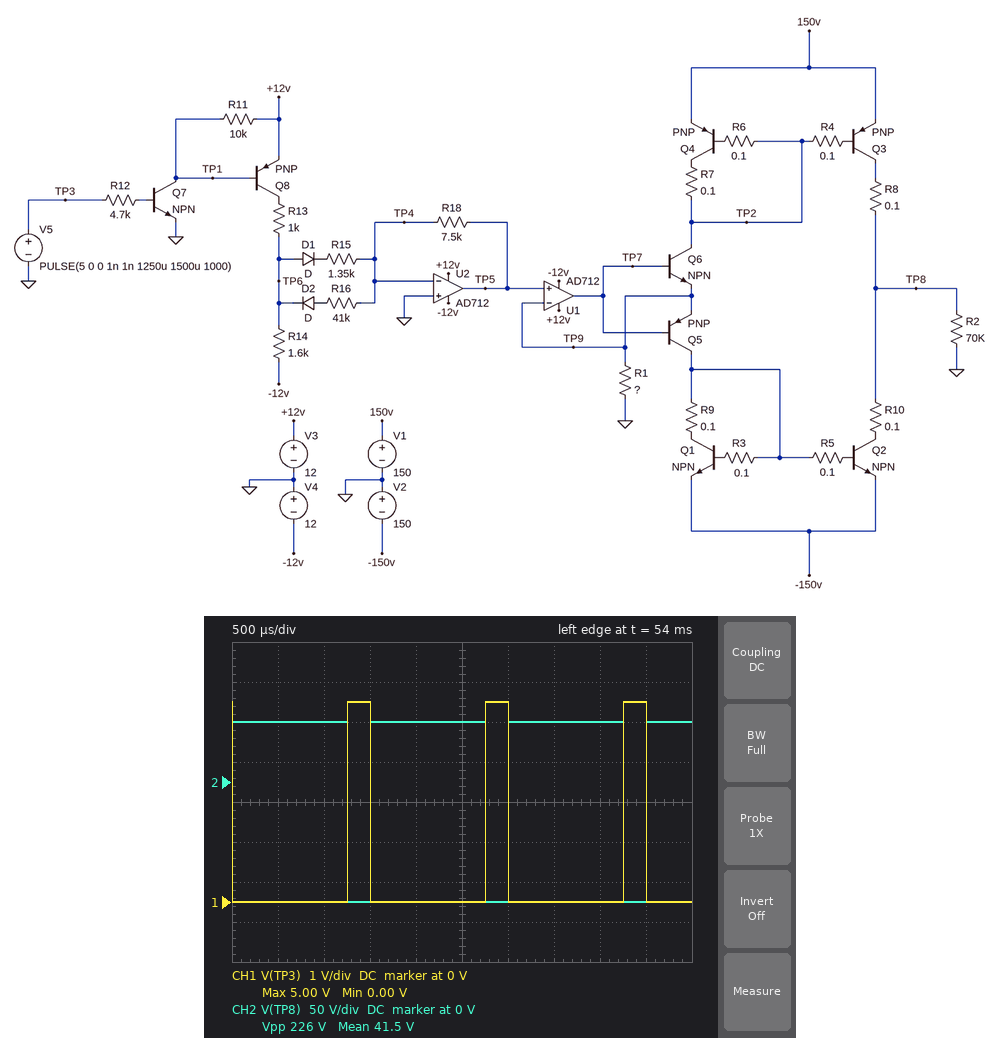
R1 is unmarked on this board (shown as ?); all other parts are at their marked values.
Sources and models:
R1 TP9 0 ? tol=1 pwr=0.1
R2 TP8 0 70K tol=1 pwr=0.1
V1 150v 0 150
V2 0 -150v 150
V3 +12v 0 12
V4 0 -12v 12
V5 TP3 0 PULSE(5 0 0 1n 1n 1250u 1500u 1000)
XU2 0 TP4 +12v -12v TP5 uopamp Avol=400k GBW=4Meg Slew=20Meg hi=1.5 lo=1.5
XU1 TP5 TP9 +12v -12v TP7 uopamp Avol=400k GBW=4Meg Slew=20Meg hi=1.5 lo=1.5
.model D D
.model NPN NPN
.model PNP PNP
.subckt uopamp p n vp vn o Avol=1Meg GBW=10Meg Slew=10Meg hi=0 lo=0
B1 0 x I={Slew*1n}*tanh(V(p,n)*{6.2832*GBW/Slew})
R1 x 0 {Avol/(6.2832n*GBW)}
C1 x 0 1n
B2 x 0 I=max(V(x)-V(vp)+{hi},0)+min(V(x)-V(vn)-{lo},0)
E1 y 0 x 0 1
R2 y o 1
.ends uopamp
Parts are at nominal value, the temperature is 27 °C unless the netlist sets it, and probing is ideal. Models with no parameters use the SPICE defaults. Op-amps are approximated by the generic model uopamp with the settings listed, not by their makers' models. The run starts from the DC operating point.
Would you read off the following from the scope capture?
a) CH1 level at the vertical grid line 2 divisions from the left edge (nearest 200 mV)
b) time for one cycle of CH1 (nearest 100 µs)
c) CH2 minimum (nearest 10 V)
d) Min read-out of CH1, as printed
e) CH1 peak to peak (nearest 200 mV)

0 V
1.5 ms
-150 V
0.00 V
5.0 V
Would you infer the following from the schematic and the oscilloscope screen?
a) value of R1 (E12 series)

1.8 kΩ
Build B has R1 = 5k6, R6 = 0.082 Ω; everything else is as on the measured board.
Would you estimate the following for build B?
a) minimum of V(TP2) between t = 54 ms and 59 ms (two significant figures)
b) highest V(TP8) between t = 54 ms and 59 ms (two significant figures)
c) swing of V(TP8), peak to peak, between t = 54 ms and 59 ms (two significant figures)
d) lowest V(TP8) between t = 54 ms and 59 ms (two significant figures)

150 V
24 V
120 V
-97 V
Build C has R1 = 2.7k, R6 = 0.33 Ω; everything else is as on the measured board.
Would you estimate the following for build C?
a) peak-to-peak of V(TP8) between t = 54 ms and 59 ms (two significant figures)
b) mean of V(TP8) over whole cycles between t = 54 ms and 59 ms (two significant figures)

200 V
17 V
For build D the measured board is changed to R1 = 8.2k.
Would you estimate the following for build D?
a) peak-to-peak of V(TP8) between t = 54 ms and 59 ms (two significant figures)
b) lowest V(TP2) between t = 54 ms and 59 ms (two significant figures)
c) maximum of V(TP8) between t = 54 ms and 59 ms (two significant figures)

83 V
150 V
17 V
